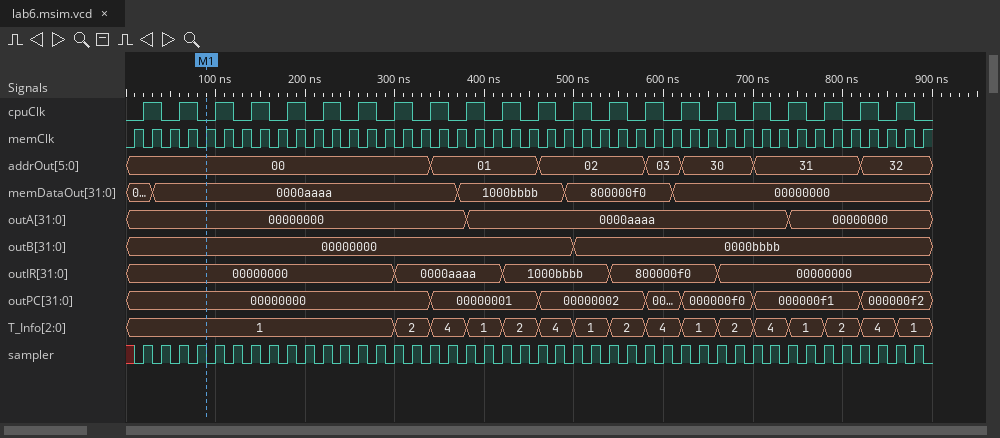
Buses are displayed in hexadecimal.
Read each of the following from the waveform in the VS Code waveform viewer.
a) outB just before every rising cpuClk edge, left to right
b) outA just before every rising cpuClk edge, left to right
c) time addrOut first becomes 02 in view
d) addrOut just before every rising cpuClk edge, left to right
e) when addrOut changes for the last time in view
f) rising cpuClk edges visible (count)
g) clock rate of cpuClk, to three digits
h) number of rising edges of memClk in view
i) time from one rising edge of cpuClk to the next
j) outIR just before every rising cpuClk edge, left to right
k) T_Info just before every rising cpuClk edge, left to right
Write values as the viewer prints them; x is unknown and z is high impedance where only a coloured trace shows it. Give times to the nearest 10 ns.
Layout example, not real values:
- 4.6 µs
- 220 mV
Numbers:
- 00000000, 00000000, 00000000, 00000000, 00000000, 00000000, 00000000, 00000000, 00000000, 00000000, 00000000, 00000000, 00000000, 0000bbbb, 0000bbbb, 0000bbbb, 0000bbbb, 0000bbbb, 0000bbbb, 0000bbbb, 0000bbbb, 0000bbbb
- 00000000, 00000000, 00000000, 00000000, 00000000, 00000000, 00000000, 00000000, 00000000, 00000000, 0000aaaa, 0000aaaa, 0000aaaa, 0000aaaa, 0000aaaa, 0000aaaa, 0000aaaa, 0000aaaa, 0000aaaa, 00000000, 00000000, 00000000
- 460 ns
- 00, 00, 00, 00, 00, 00, 00, 00, 00, 01, 01, 01, 02, 02, 02, 03, 30, 30, 31, 31, 31, 32
- 820 ns
- 22
- 25.0 MHz
- 45
- 40 ns
- 00000000, 00000000, 00000000, 00000000, 00000000, 00000000, 00000000, 00000000, 0000aaaa, 0000aaaa, 0000aaaa, 1000bbbb, 1000bbbb, 1000bbbb, 800000f0, 800000f0, 800000f0, 00000000, 00000000, 00000000, 00000000, 00000000
- 1, 1, 1, 1, 1, 1, 1, 1, 2, 4, 1, 2, 4, 1, 2, 4, 1, 2, 4, 1, 2, 4
